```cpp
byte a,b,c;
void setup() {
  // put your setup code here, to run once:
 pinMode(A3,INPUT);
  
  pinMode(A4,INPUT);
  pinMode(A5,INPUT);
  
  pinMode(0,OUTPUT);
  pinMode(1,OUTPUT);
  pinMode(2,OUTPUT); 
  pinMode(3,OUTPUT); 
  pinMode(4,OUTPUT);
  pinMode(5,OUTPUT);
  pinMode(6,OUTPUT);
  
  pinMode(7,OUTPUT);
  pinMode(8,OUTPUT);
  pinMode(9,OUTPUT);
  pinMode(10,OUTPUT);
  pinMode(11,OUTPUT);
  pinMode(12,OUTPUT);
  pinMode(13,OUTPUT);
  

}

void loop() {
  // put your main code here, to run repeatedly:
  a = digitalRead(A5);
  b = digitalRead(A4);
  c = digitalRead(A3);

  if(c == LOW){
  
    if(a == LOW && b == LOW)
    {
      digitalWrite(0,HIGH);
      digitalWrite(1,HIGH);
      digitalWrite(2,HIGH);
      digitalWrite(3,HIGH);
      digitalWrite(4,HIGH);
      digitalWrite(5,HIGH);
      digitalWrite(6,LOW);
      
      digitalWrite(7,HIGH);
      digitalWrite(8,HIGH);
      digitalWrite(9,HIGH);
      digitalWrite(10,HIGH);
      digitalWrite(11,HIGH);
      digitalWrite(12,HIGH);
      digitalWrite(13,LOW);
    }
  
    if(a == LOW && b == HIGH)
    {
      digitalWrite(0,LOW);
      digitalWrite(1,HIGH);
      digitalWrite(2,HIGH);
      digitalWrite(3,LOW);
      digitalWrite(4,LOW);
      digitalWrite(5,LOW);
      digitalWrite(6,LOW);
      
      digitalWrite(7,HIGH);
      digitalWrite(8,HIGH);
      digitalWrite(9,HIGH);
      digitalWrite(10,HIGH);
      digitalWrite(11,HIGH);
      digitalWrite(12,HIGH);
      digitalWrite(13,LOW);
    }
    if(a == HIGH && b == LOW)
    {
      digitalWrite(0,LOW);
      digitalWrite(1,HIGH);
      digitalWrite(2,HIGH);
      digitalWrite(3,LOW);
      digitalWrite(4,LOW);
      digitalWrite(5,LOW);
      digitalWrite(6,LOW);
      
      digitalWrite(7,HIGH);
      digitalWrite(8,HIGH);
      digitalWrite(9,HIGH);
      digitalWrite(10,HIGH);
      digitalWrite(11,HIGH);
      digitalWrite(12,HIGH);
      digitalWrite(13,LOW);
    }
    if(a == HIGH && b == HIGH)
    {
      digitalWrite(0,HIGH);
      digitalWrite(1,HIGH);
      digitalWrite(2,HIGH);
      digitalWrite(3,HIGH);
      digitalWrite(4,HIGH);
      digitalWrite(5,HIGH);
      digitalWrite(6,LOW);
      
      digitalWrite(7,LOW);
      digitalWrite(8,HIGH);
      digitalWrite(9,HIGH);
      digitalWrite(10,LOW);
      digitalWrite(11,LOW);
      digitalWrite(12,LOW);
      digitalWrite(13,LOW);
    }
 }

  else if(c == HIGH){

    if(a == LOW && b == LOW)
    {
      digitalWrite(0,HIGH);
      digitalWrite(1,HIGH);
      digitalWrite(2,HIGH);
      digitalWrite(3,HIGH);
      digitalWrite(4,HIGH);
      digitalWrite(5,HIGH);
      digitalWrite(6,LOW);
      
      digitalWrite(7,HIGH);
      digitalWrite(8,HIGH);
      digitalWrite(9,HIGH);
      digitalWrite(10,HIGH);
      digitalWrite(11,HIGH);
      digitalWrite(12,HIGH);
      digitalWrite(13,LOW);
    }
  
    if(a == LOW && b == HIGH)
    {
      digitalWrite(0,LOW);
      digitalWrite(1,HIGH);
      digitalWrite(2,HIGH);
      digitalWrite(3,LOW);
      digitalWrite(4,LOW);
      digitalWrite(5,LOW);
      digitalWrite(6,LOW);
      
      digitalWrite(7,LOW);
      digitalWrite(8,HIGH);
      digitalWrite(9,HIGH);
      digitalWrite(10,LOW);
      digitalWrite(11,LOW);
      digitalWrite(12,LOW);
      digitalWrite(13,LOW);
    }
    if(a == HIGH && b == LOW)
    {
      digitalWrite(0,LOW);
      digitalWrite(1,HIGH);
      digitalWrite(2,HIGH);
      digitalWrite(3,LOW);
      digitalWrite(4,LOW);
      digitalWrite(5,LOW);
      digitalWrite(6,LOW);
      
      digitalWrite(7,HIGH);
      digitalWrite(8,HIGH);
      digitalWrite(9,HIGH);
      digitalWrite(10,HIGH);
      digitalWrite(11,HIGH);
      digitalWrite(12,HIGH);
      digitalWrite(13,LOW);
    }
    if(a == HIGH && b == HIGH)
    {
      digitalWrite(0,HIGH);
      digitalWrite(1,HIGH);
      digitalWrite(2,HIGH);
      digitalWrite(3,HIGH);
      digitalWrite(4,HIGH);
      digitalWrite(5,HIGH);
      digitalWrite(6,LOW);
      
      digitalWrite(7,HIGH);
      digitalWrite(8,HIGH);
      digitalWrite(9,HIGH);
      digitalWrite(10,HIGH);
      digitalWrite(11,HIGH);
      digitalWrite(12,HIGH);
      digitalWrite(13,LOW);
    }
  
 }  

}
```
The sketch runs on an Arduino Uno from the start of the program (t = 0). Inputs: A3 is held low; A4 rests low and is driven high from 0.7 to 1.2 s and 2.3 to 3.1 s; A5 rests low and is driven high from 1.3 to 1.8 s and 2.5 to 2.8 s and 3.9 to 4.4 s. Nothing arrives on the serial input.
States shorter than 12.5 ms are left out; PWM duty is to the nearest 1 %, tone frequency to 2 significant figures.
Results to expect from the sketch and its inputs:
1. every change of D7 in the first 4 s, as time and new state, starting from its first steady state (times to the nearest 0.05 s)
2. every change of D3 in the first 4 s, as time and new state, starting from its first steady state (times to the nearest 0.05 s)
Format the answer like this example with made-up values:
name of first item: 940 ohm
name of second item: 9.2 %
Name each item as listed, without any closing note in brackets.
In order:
every change of D7 in the first 4 s, as time and new state, starting from its first steady state: 0 s high; 2.5 s low; 2.8 s high
every change of D3 in the first 4 s, as time and new state, starting from its first steady state: 0 s high; 0.7 s low; 1.2 s high; 1.3 s low; 1.8 s high; 2.3 s low; 2.5 s high; 2.8 s low; 3.1 s high; 3.9 s low
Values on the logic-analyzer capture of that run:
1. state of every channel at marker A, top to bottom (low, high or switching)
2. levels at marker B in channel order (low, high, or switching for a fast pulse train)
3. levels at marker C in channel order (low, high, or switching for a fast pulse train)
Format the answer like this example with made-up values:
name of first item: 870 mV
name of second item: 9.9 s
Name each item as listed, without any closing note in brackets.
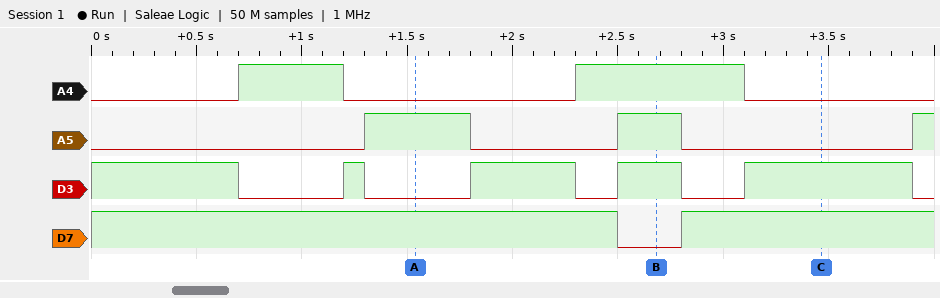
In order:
state of every channel at marker A, top to bottom: A4 low, A5 high, D3 low, D7 high
levels at marker B in channel order: A4 high, A5 high, D3 high, D7 low
levels at marker C in channel order: A4 low, A5 low, D3 high, D7 high
